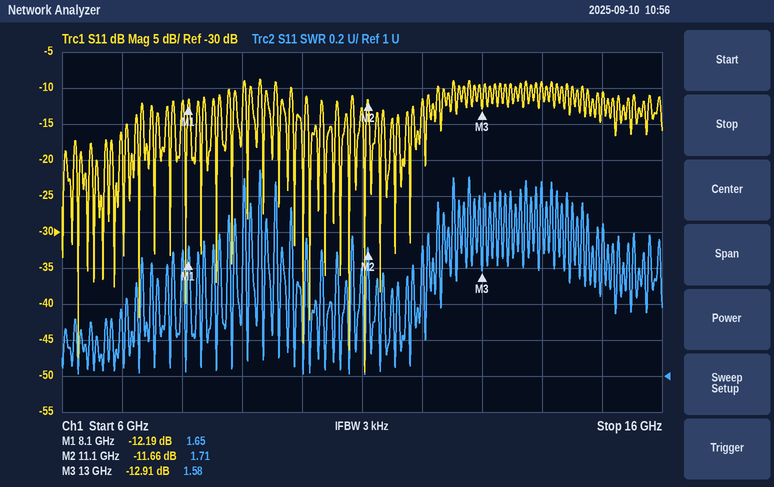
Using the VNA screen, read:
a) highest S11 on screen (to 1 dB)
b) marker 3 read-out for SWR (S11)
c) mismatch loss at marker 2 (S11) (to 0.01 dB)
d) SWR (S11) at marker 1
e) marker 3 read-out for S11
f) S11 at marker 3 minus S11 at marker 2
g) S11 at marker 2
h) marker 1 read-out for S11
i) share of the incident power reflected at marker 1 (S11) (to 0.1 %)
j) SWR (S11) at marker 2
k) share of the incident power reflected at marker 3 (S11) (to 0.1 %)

-9 dB
1.58
0.31 dB
1.65
-12.91 dB
-1.25 dB
-11.66 dB
-12.19 dB
6.0 %
1.71
5.1 %
